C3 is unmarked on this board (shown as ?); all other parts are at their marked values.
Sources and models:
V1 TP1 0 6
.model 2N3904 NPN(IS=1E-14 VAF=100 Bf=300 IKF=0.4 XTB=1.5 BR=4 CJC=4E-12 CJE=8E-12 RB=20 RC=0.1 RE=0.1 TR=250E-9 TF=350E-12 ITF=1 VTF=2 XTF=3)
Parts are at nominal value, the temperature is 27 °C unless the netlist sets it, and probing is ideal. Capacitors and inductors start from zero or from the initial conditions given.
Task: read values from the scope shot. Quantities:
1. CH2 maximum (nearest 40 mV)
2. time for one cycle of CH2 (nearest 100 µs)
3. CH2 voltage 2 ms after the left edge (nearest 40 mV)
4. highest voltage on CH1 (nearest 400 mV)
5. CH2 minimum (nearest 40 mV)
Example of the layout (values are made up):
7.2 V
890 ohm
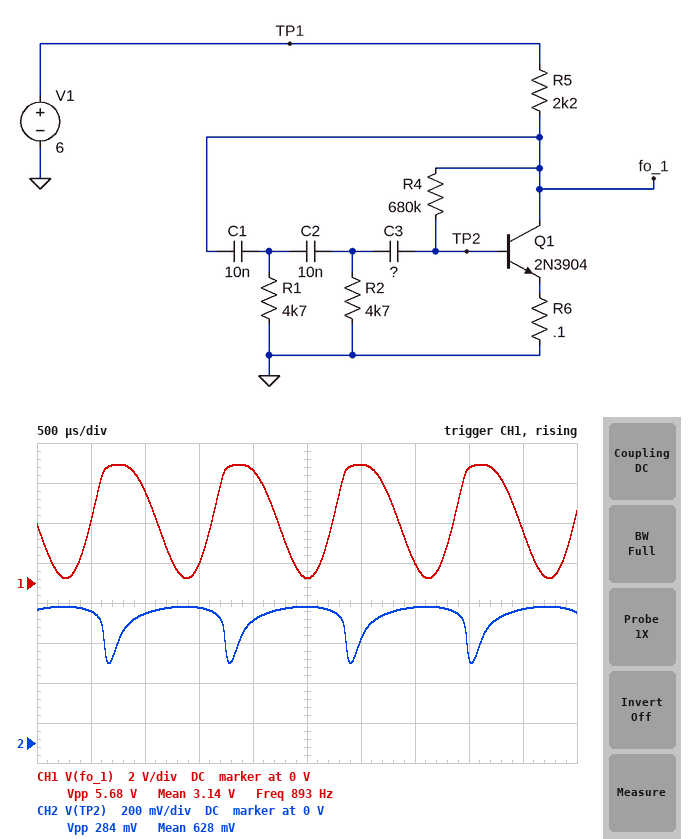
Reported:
680 mV
1.1 ms
600 mV
6.0 V
400 mV
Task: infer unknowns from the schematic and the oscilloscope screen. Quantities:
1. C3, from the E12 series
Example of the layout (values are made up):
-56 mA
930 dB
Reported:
12 nF
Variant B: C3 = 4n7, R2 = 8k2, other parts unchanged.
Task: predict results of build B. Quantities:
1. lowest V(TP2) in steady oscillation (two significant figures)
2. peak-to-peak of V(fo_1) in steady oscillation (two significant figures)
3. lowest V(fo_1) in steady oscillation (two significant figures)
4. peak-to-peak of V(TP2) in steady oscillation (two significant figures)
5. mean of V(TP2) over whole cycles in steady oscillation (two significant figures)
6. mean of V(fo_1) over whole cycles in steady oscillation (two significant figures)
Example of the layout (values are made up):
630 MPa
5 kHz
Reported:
270 mV
5.8 V
120 mV
410 mV
600 mV
3.4 V
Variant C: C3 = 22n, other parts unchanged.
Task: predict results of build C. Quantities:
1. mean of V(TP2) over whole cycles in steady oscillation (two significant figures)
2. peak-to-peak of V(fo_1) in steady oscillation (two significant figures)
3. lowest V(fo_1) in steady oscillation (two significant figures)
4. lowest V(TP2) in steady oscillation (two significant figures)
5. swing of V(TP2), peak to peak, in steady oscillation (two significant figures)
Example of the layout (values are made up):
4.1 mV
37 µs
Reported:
640 mV
5.3 V
580 mV
500 mV
180 mV
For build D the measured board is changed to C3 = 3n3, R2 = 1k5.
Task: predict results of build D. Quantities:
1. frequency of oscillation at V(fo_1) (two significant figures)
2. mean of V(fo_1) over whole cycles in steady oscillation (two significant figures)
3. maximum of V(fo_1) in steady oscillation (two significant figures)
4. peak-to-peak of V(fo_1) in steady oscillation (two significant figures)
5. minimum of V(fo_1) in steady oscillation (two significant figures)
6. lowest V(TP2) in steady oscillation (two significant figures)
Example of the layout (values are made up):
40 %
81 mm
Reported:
2.1 kHz
3.3 V
5.8 V
5.4 V
410 mV
470 mV
